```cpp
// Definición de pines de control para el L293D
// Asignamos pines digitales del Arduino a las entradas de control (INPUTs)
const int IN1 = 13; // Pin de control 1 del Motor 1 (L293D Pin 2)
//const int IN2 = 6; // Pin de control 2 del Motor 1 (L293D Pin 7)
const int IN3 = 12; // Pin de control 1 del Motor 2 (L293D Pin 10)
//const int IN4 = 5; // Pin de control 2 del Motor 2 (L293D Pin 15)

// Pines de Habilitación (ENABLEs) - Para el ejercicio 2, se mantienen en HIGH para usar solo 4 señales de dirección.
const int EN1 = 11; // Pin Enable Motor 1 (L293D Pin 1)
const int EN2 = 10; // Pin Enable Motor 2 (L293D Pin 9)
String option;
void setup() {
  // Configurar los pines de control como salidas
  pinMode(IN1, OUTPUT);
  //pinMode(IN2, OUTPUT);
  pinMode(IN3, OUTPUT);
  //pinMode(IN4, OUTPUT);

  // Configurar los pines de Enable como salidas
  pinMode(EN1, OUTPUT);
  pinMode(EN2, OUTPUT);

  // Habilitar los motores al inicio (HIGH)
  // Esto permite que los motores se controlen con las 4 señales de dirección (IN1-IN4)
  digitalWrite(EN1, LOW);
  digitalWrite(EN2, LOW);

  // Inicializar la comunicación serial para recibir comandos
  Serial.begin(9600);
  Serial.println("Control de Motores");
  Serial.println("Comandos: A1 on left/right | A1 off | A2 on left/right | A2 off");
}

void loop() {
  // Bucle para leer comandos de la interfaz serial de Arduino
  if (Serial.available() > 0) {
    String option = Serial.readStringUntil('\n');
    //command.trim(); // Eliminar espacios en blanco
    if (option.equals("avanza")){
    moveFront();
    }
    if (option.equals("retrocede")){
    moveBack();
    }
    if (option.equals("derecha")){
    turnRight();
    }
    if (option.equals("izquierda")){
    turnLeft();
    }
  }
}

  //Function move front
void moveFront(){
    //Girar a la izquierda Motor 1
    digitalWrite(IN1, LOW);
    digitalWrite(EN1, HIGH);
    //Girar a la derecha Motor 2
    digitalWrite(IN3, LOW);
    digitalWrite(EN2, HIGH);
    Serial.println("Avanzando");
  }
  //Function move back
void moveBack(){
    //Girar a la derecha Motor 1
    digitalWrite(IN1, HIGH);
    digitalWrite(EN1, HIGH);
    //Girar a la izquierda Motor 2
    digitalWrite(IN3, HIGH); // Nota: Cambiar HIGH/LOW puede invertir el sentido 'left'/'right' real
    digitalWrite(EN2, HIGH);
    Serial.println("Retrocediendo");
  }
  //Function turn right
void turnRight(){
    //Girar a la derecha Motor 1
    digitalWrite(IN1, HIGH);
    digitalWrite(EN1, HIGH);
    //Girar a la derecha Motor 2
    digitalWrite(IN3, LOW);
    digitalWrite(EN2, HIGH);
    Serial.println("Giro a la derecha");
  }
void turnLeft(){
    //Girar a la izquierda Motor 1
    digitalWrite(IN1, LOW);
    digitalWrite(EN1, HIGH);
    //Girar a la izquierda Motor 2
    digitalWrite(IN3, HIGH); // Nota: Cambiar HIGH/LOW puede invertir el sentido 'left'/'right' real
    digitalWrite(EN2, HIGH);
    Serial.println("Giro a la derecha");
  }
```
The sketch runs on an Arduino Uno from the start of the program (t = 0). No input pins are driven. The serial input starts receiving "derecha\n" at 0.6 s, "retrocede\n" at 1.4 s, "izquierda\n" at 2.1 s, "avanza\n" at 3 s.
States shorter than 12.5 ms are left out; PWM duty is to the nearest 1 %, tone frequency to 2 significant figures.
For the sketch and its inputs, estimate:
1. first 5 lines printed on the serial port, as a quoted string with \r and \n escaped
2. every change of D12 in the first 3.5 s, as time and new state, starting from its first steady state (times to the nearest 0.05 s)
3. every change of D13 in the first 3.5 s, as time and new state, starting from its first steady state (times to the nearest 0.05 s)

"Control de Motores\r\nComandos: A1 on left/right | A1 off | A2 on left/right | A2 off\r\nGiro a la derecha\r\nRetrocediendo\r\nGiro a la derecha\r\n"
0 s low; 1.4 s high; 3 s low
0 s low; 0.6 s high; 2.1 s low
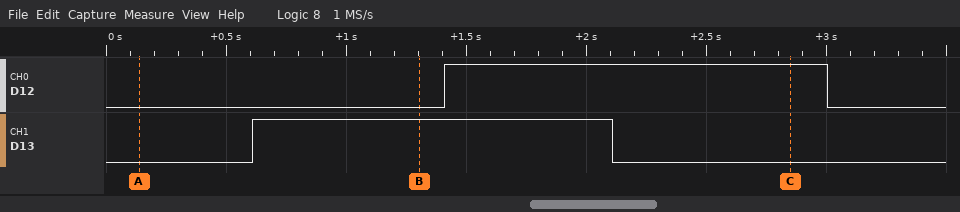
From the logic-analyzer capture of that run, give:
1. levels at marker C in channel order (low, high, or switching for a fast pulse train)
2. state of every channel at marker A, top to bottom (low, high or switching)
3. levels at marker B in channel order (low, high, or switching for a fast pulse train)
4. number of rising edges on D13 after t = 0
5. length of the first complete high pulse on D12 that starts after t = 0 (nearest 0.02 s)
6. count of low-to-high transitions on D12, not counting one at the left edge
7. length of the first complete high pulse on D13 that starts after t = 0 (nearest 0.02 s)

D12 high, D13 low
D12 low, D13 low
D12 low, D13 high
1
1.60 s
1
1.50 s
